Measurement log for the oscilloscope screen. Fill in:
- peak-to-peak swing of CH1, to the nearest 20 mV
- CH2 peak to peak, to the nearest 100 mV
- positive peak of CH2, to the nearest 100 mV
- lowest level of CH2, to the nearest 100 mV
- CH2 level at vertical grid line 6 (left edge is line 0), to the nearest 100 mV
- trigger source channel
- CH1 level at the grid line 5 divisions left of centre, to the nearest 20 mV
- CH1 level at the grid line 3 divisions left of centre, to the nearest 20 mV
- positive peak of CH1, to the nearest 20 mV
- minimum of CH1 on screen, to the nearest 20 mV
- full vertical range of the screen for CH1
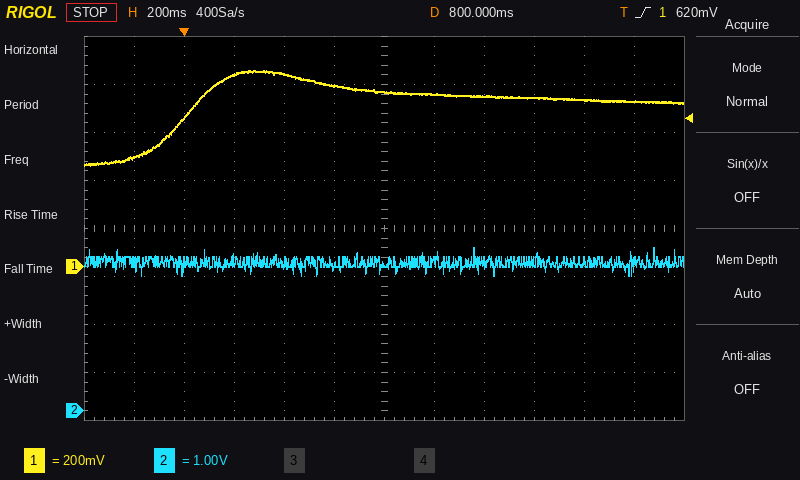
400 mV
600 mV
3.4 V
2.8 V
3.1 V
CH1
460 mV
800 mV
820 mV
420 mV
1.6 V
